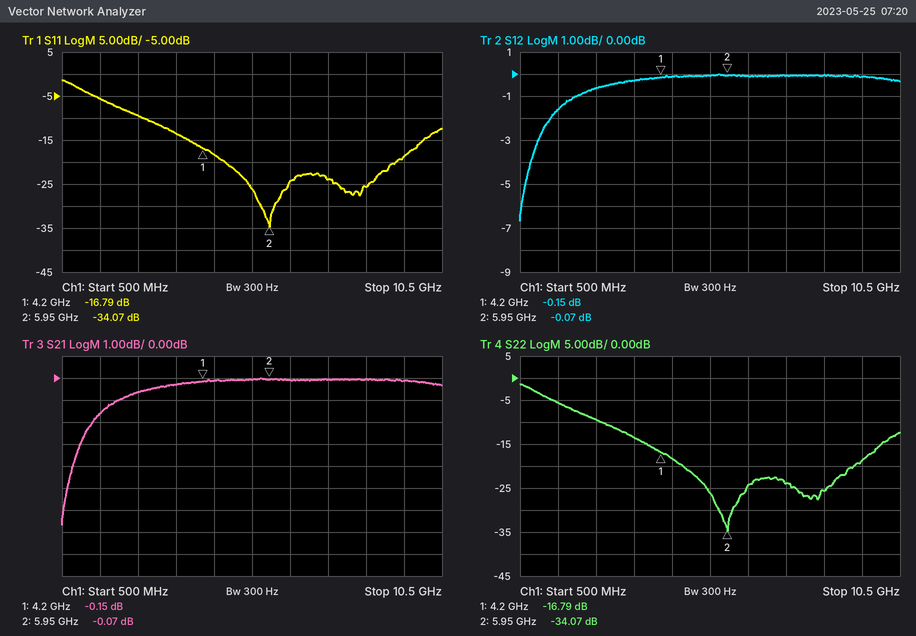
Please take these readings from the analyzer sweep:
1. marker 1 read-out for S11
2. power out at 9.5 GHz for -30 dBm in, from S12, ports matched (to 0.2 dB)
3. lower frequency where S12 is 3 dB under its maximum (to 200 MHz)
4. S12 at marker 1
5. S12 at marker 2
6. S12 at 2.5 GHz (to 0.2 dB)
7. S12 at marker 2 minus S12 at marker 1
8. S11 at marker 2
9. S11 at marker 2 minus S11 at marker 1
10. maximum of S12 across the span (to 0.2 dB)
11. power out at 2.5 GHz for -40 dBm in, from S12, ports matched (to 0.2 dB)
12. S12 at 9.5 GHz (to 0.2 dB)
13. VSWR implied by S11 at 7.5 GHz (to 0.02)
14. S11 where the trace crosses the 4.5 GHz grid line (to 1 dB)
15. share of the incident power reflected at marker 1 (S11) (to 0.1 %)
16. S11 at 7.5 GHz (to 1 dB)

-16.79 dB
-30.2 dBm
1.0 GHz
-0.15 dB
-0.07 dB
-0.6 dB
0.08 dB
-34.07 dB
-17.28 dB
0.0 dB
-40.6 dBm
-0.2 dB
1.14
-18 dB
2.1 %
-24 dB
